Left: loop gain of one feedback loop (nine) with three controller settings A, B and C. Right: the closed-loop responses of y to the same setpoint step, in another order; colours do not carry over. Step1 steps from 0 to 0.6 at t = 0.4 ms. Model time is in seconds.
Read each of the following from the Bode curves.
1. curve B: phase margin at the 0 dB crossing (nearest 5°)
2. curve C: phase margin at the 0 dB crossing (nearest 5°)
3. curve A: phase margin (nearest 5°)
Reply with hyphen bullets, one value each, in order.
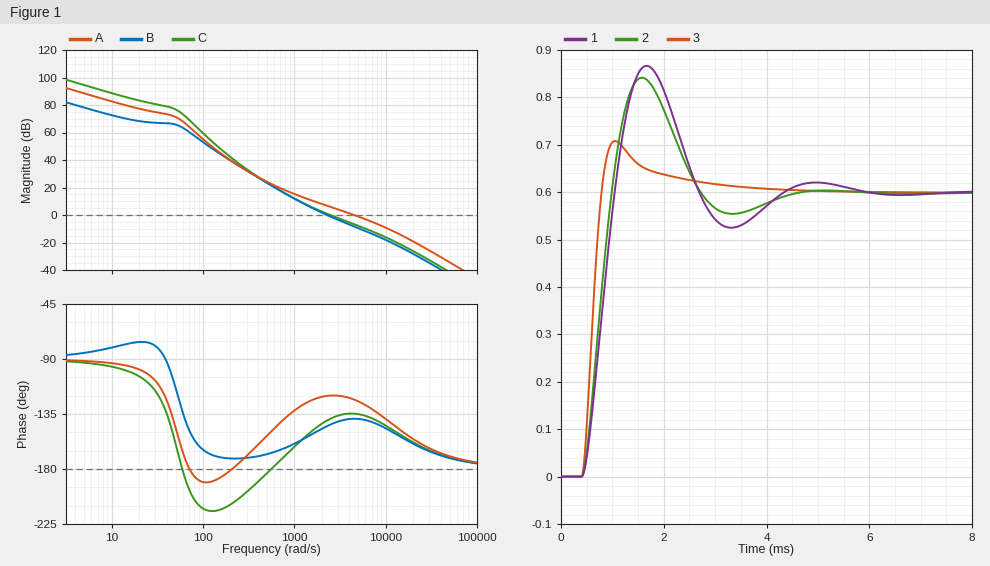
- 35°
- 40°
- 55°
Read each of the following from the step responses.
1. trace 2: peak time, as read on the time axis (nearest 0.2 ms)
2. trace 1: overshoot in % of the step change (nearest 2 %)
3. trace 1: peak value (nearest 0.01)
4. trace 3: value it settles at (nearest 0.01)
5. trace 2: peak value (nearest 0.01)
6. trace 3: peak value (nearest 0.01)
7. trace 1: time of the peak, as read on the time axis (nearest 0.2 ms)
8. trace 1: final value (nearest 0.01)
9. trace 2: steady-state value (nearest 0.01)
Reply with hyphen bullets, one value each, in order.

- 1.6 ms
- 44 %
- 0.87
- 0.60
- 0.84
- 0.71
- 1.6 ms
- 0.60
- 0.60
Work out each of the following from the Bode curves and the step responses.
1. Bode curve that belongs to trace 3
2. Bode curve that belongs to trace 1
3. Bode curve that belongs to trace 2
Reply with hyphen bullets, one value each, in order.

- A
- B
- C
